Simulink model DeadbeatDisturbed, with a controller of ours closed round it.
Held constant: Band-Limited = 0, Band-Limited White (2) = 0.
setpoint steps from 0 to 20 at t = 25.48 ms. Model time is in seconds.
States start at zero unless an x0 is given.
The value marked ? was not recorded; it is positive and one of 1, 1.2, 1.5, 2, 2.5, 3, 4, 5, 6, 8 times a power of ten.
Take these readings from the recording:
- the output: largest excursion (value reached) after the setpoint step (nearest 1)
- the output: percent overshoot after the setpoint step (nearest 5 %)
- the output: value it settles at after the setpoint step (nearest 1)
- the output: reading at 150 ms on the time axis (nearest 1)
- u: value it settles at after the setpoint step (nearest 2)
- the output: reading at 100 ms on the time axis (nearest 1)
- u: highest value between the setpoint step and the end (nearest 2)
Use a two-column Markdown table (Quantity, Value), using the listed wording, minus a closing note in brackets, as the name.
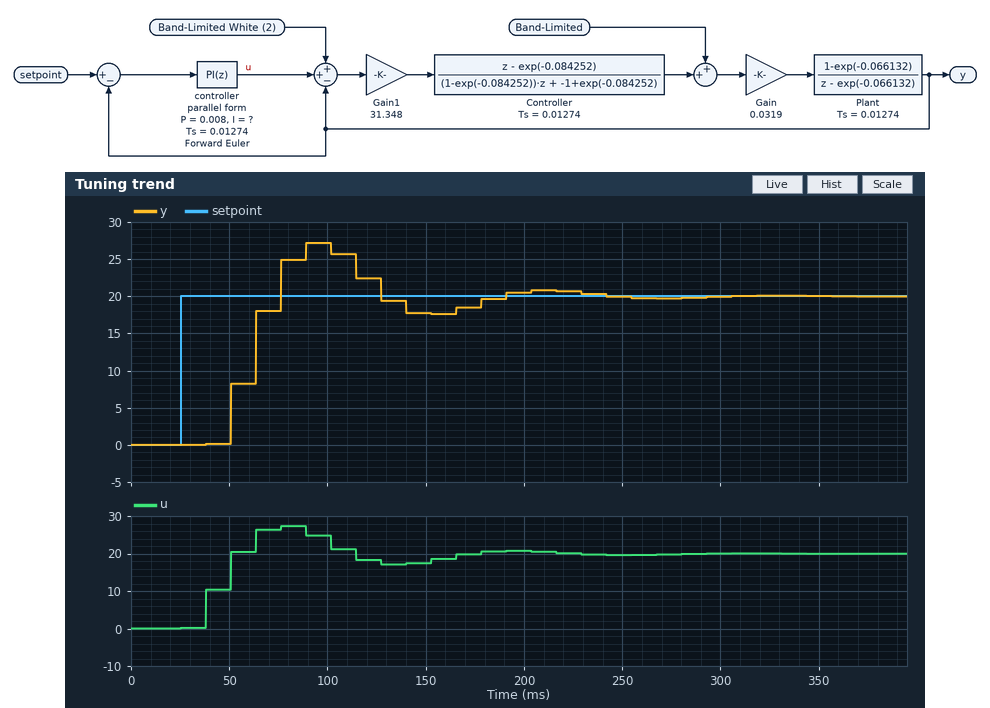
| Quantity | Value |
|---|---|
| the output: largest excursion (value reached) after the setpoint step | 27 |
| the output: percent overshoot after the setpoint step | 35 % |
| the output: value it settles at after the setpoint step | 20 |
| the output: reading at 150 ms on the time axis | 18 |
| u: value it settles at after the setpoint step | 20 |
| the output: reading at 100 ms on the time axis | 27 |
| u: highest value between the setpoint step and the end | 28 |
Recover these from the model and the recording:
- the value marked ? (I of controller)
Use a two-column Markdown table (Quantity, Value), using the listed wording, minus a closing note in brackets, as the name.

| Quantity | Value |
|---|---|
| the value marked ? | 40 |
